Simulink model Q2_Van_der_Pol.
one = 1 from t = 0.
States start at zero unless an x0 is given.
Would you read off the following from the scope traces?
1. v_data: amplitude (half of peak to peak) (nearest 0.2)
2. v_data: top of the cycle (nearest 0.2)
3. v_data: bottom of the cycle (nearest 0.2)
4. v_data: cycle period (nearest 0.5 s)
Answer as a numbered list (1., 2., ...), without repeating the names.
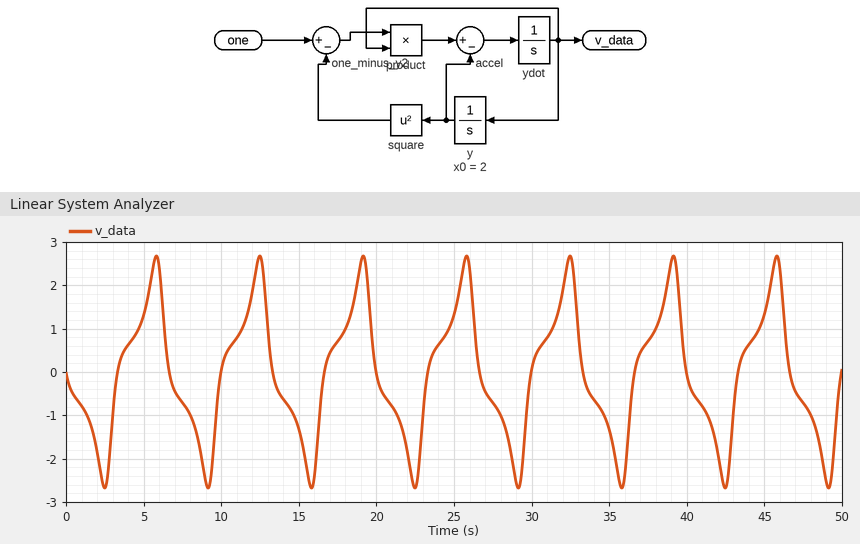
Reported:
1. 2.6
2. 2.6
3. -2.6
4. 6.5 s
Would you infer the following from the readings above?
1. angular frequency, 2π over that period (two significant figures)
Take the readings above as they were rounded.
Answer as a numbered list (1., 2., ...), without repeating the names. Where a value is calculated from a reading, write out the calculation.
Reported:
1. 2π / 6.5 = 0.97 rad/s
